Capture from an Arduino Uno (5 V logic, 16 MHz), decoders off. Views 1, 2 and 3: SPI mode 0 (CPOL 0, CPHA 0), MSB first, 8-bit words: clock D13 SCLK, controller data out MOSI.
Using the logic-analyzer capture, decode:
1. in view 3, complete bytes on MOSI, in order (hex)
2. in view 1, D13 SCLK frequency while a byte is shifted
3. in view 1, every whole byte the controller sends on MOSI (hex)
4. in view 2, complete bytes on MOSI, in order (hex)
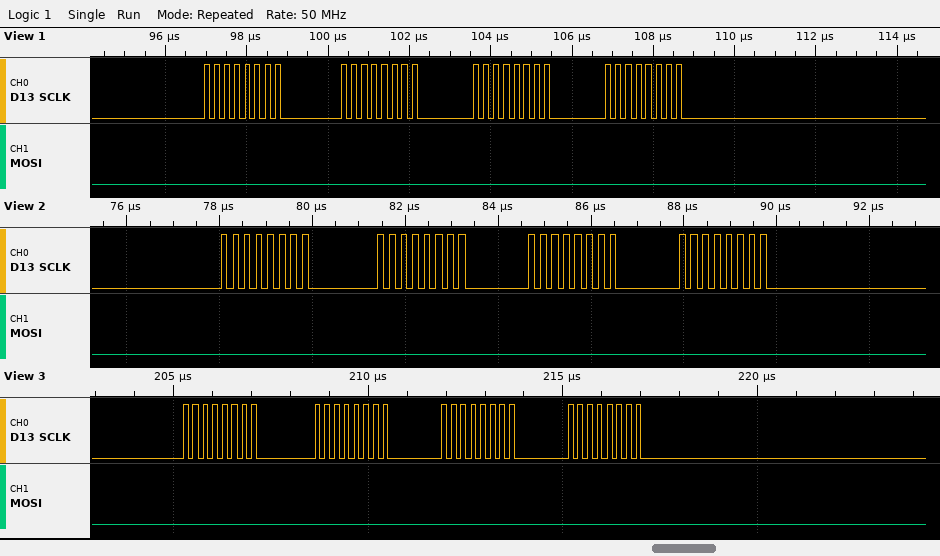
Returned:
00 00 00 00
4 MHz
0x00 0x00 0x00 0x00
0x00 0x00 0x00 0x00
